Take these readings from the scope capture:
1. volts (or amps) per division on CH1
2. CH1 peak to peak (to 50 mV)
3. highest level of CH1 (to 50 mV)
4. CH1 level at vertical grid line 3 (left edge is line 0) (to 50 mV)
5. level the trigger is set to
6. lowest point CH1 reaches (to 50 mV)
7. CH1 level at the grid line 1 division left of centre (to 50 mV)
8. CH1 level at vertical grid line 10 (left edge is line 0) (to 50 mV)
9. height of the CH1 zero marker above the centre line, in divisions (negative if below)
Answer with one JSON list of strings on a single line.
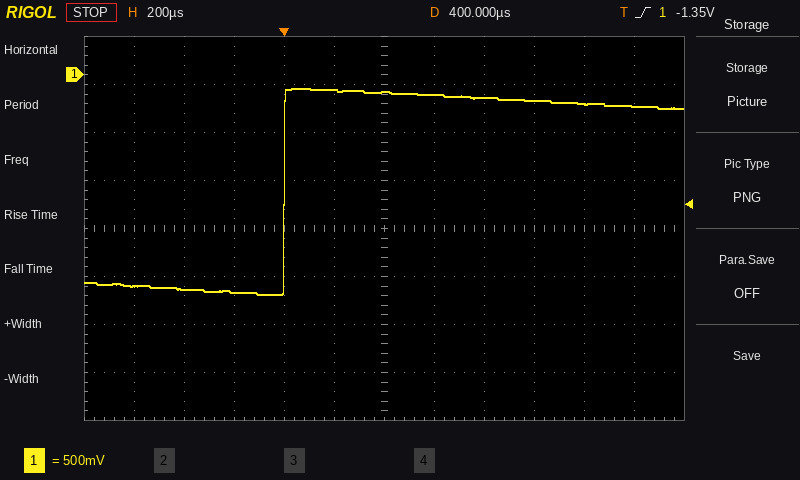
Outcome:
["500 mV", "2.15 V", "-150 mV", "-2.25 V", "-1.35 V", "-2.30 V", "-150 mV", "-300 mV", "+3.2 div"]
